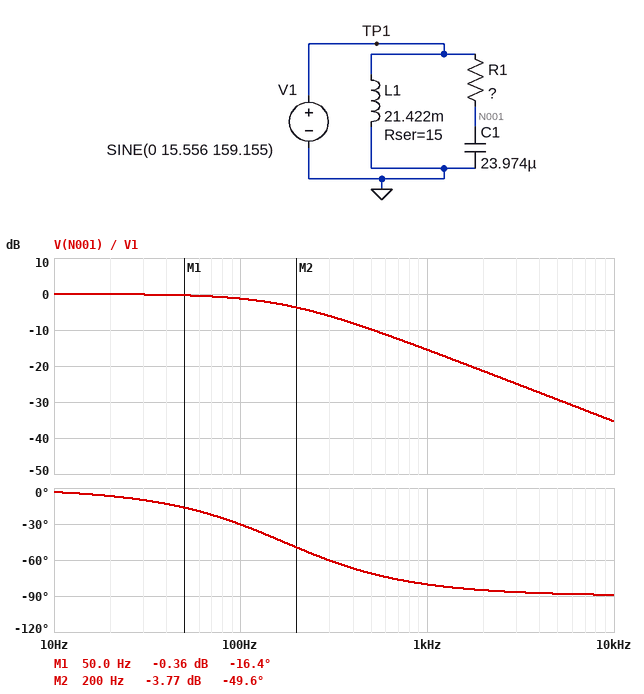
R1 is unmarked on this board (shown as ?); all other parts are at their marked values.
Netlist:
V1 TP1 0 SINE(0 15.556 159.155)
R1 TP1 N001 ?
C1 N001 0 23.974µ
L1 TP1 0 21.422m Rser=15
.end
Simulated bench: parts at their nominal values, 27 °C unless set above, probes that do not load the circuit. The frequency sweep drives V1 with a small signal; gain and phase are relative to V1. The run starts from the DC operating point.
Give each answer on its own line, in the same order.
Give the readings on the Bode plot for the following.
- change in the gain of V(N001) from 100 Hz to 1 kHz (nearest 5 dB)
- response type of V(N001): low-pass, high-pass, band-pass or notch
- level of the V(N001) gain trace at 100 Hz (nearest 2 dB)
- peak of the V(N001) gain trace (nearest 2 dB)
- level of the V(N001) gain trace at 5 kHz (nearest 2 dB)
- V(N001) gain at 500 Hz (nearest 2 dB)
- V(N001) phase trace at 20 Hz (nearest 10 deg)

-15 dB
low-pass
-2 dB
0 dB
-30 dB
-10 dB
-10 deg
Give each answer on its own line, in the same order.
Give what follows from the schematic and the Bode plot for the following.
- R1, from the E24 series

39 Ω
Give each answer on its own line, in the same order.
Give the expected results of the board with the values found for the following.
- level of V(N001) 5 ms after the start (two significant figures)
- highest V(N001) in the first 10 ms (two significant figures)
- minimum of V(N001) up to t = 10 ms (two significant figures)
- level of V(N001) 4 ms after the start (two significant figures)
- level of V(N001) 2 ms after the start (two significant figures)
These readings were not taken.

-10 V
12 V
-11 V
-1.1 V
12 V
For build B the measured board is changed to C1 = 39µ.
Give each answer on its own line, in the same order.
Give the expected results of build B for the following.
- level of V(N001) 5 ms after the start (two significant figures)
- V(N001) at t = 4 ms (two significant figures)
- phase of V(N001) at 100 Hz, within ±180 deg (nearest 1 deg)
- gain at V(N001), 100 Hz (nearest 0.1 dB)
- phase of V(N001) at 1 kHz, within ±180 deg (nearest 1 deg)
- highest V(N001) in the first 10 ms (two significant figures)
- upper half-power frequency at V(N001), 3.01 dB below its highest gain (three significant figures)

-6.3 V
1.6 V
-44 deg
-2.8 dB
-84 deg
9.9 V
105 Hz
